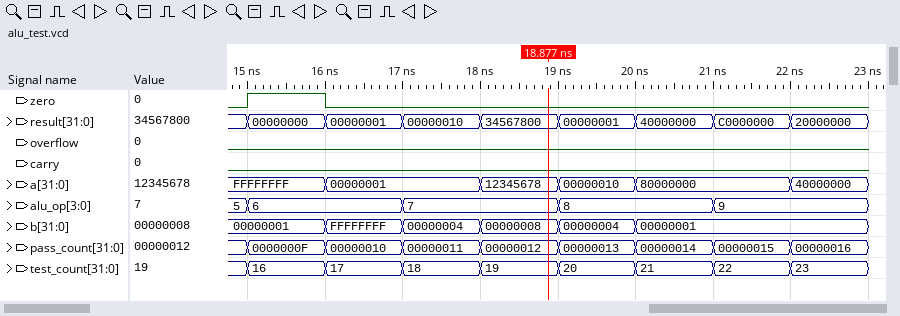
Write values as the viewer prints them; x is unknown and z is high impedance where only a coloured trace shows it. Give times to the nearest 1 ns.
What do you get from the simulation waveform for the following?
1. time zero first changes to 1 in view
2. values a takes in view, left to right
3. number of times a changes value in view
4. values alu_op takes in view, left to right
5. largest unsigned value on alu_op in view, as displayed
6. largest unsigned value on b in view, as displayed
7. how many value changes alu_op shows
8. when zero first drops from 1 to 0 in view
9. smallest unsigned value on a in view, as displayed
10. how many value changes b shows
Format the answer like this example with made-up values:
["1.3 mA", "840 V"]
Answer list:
["15 ns", "FFFFFFFF, 00000001, 12345678, 00000010, 80000000, 40000000", "5", "5, 6, 7, 8, 9", "9", "FFFFFFFF", "4", "16 ns", "00000001", "5"]
